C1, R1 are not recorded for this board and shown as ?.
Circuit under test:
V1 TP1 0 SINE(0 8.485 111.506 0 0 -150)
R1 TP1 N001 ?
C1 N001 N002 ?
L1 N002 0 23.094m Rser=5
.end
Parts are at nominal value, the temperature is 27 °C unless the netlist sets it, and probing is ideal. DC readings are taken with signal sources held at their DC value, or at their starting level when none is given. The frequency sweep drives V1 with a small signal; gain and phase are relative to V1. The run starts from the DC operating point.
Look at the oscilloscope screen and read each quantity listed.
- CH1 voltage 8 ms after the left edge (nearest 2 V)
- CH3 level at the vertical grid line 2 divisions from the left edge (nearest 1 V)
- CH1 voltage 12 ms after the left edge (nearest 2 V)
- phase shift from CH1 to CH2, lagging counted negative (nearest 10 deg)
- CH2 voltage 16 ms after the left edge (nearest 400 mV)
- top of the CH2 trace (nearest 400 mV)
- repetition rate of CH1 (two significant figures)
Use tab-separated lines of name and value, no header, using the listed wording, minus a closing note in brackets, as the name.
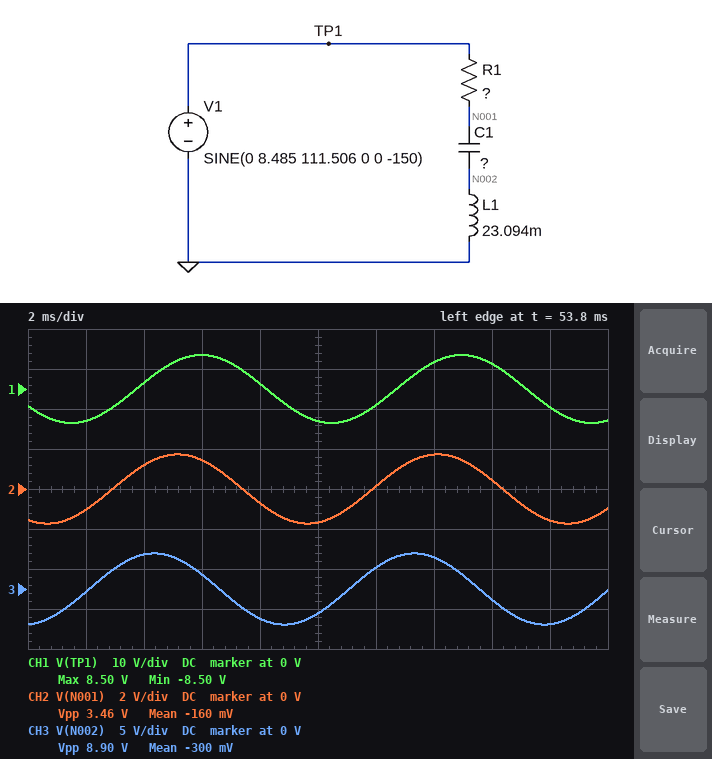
CH1 voltage 8 ms after the left edge	2 V
CH3 level at the vertical grid line 2 divisions from the left edge	4 V
CH1 voltage 12 ms after the left edge	-4 V
phase shift from CH1 to CH2, lagging counted negative	30 deg
CH2 voltage 16 ms after the left edge	400 mV
top of the CH2 trace	1.6 V
repetition rate of CH1	110 Hz
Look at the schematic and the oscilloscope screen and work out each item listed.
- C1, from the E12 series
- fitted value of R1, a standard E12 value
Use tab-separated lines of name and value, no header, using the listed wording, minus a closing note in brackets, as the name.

C1, from the E12 series	120 µF
fitted value of R1, a standard E12 value	27 Ω
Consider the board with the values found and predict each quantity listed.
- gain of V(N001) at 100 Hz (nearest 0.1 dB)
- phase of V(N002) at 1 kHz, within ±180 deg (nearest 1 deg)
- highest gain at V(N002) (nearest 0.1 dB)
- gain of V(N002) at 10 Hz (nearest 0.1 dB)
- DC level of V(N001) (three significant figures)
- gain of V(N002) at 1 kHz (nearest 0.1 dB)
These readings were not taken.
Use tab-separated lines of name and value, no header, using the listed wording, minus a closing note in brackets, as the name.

gain of V(N001) at 100 Hz	-15.9 dB
phase of V(N002) at 1 kHz, within ±180 deg	11 deg
highest gain at V(N002)	0 dB
gain of V(N002) at 10 Hz	-28.3 dB
DC level of V(N001)	-4.24 V
gain of V(N002) at 1 kHz	-0.1 dB
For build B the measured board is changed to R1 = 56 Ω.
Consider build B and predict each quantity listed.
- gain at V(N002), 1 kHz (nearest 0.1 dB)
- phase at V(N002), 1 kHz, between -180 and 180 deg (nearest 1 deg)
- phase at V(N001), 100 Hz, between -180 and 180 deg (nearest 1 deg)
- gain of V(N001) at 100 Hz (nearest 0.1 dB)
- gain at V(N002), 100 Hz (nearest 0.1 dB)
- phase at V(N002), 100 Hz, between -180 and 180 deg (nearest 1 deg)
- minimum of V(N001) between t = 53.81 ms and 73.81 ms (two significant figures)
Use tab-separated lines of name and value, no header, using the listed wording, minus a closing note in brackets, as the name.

gain at V(N002), 1 kHz	-0.6 dB
phase at V(N002), 1 kHz, between -180 and 180 deg	21 deg
phase at V(N001), 100 Hz, between -180 and 180 deg	13 deg
gain of V(N001) at 100 Hz	-21.5 dB
gain at V(N002), 100 Hz	-12.0 dB
phase at V(N002), 100 Hz, between -180 and 180 deg	70 deg
minimum of V(N001) between t = 53.81 ms and 73.81 ms	-920 mV
